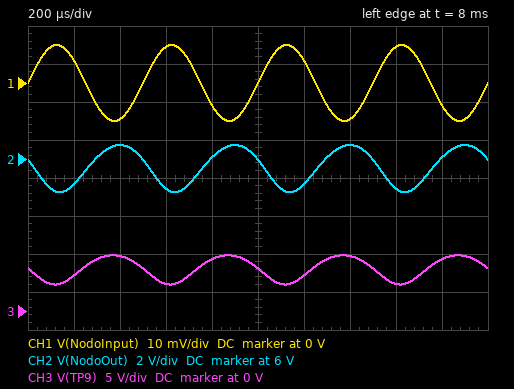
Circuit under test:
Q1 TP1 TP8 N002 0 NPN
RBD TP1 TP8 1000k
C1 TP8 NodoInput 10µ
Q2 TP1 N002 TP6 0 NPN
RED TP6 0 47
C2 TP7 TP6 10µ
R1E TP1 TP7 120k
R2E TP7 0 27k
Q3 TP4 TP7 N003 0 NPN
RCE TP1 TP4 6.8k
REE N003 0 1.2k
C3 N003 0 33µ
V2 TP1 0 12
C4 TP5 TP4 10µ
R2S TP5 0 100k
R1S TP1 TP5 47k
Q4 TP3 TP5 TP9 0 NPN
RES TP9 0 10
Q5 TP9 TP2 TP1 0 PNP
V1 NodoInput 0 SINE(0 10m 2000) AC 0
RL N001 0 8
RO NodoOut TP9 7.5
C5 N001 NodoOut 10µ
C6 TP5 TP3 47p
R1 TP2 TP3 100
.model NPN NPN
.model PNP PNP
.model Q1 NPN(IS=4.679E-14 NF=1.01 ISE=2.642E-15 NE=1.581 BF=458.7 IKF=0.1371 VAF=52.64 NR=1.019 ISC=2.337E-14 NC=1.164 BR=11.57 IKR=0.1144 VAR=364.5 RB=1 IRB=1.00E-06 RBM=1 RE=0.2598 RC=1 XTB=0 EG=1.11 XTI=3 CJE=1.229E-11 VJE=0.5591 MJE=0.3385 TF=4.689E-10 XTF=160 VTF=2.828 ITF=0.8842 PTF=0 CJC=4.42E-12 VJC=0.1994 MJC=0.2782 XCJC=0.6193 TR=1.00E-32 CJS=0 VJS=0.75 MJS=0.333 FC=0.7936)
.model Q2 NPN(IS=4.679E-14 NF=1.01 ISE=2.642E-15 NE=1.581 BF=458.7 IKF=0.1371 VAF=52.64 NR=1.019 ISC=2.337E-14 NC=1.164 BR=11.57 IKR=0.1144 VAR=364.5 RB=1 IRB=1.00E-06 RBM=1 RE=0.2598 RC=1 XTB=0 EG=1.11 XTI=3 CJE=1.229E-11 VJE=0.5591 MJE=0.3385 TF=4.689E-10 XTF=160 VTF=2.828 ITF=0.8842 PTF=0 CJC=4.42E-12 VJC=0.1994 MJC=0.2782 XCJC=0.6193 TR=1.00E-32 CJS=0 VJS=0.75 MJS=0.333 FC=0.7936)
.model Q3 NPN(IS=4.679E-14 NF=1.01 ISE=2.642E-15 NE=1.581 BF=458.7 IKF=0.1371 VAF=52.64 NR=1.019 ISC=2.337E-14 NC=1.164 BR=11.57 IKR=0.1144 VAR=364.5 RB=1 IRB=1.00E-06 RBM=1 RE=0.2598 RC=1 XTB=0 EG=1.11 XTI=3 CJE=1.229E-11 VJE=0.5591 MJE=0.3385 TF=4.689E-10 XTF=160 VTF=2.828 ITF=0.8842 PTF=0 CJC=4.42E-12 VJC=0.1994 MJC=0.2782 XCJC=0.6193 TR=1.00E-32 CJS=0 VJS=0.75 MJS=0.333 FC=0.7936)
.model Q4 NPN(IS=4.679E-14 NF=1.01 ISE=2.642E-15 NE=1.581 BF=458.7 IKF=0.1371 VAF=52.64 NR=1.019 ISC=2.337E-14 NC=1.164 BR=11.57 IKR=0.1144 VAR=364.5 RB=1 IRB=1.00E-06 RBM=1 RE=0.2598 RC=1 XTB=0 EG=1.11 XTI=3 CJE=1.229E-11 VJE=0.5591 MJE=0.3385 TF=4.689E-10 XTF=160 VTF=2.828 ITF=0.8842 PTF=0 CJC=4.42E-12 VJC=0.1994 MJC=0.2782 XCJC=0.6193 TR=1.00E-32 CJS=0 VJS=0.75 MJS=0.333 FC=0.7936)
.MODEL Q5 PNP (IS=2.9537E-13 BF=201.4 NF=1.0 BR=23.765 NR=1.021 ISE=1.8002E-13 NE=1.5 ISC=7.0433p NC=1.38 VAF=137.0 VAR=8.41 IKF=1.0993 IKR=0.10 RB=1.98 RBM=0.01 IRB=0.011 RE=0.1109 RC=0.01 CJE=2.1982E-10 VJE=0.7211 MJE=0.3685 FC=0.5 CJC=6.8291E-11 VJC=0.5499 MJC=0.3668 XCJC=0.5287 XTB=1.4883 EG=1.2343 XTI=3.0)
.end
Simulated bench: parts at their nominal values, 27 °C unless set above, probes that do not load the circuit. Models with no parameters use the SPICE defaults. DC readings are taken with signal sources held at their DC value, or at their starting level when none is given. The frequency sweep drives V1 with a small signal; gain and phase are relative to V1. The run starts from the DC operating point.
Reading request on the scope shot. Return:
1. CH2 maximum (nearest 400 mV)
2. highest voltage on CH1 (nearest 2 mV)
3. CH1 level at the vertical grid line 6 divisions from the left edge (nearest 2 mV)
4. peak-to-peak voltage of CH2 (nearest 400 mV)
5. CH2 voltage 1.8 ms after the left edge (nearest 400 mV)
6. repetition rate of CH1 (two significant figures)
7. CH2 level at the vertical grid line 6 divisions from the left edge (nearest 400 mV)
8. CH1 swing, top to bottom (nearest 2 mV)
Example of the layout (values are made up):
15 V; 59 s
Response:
6.8 V; 10 mV; 6 mV; 2.4 V; 6.0 V; 2.0 kHz; 4.8 V; 20 mV
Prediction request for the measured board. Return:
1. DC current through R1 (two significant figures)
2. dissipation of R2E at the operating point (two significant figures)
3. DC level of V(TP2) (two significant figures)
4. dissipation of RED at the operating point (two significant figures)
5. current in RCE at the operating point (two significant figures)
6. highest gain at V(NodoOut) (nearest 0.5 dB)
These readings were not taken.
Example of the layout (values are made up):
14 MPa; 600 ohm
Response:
5.5 mA; 150 µW; 11 V; 240 mW; 1.0 mA; 44.5 dB
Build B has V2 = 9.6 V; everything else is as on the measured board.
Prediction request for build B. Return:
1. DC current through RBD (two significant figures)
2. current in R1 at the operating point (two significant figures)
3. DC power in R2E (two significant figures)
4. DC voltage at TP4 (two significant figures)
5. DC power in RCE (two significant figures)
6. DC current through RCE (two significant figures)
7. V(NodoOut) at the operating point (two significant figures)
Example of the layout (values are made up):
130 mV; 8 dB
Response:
5.4 µA; 4.3 mA; 96 µW; 4.9 V; 3.3 mW; 700 µA; 4.3 V
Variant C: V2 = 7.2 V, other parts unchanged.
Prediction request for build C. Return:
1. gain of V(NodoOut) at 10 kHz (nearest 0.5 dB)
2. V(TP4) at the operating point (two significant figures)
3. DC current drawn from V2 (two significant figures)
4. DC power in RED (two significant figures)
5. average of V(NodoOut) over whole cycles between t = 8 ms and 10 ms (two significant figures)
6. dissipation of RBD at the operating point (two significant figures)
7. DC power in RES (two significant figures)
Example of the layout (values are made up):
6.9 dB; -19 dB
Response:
32.0 dB; 4.5 V; 350 mA; 70 mW; 3.1 V; 14 µW; 970 mW
